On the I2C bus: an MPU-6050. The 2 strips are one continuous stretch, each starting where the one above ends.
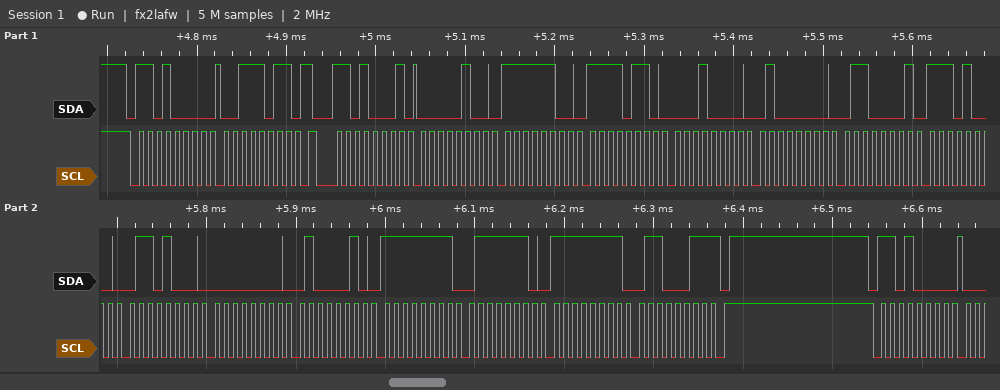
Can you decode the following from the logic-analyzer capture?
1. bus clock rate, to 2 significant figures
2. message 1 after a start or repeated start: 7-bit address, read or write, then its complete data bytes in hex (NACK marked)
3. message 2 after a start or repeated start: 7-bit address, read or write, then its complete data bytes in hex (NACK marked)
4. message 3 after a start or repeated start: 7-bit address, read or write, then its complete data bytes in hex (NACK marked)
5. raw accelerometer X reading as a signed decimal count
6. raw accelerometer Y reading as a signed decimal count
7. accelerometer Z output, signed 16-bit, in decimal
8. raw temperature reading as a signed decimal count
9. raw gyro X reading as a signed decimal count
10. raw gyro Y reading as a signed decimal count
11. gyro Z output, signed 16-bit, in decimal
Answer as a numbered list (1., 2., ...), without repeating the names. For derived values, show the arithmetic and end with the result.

1. 100 kHz
2. 0x68 write: 3B
3. 0x68 read: 04 FC F6 10 40 61 E8 68 00 42 FF 7E FF 63 NACK
4. 0x68 write
5. 0x04FC = 1276
6. 0xF610 = -2544
7. 0x4061 = 16481
8. 0xE868 = -6040
9. 0x0042 = 66
10. 0xFF7E = -130
11. 0xFF63 = -157
